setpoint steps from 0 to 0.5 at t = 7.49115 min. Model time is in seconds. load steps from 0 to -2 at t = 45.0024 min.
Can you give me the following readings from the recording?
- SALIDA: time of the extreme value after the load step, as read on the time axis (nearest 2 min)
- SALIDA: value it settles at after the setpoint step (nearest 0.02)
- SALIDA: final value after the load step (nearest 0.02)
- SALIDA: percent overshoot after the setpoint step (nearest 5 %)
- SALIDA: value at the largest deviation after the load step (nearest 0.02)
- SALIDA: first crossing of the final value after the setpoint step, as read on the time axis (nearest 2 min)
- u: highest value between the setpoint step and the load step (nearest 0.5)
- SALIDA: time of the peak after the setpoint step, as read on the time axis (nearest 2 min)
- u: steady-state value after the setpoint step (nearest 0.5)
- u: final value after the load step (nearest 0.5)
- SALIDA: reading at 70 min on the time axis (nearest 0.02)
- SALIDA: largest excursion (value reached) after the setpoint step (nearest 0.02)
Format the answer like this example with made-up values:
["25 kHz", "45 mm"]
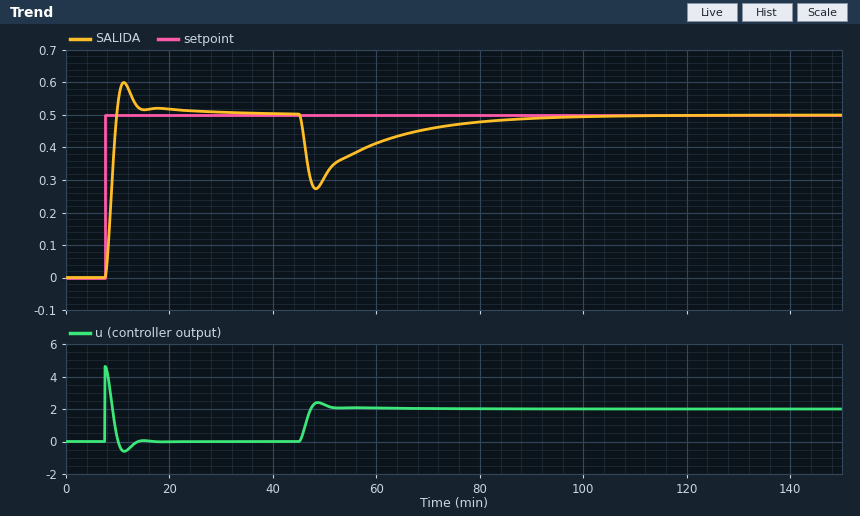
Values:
["48 min", "0.50", "0.50", "20 %", "0.28", "10 min", "4.5", "12 min", "0.0", "2.0", "0.46", "0.60"]
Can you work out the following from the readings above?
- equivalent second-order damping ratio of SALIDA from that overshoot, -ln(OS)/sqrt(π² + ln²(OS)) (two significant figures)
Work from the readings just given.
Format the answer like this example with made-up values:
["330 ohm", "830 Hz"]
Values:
["0.46"]
